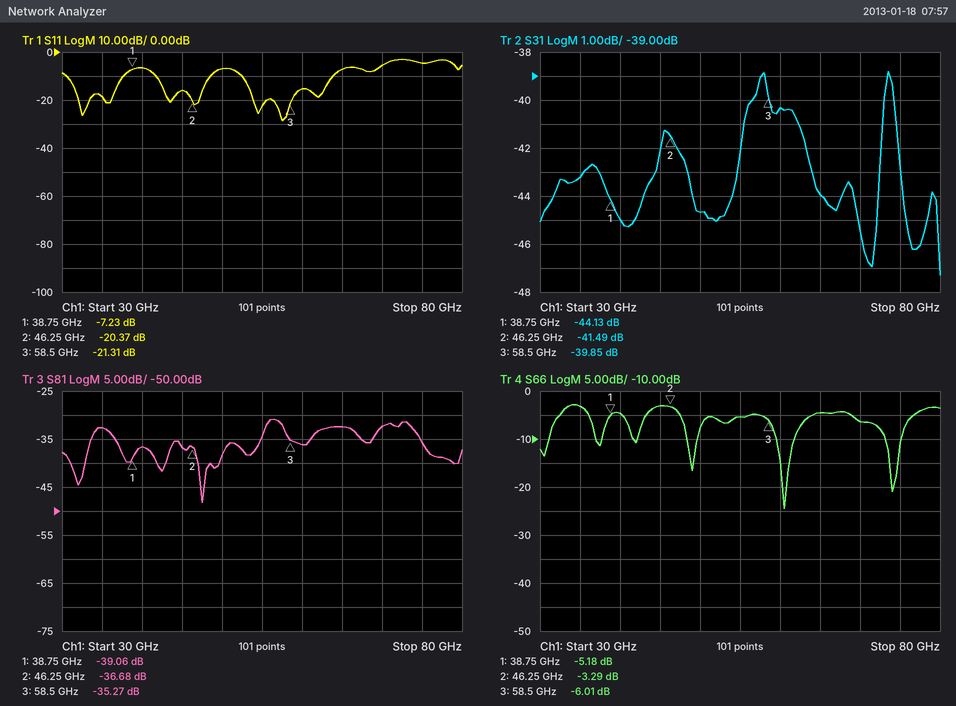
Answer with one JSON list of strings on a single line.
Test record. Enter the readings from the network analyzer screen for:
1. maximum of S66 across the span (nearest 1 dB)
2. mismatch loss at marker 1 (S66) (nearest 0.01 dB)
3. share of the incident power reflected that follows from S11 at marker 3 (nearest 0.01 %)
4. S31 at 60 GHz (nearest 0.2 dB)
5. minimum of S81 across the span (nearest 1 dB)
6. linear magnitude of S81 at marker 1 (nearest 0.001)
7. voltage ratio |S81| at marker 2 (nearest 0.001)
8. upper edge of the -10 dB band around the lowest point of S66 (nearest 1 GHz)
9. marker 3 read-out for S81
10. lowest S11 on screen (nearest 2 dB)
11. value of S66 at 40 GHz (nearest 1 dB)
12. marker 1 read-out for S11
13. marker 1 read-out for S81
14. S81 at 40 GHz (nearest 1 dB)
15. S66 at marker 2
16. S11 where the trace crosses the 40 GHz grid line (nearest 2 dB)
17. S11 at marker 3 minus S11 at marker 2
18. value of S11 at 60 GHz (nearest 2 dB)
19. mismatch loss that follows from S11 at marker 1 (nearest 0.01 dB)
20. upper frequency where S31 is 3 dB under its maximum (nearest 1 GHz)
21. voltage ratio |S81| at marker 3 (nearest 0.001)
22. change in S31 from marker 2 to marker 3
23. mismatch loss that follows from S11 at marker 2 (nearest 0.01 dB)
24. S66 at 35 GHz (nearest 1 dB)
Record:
["-3 dB", "1.57 dB", "0.74 %", "-40.4 dB", "-48 dB", "0.011", "0.015", "62 GHz", "-35.27 dB", "-28 dB", "-5 dB", "-7.23 dB", "-39.06 dB", "-37 dB", "-3.29 dB", "-6 dB", "-0.94 dB", "-16 dB", "0.91 dB", "75 GHz", "0.017", "1.64 dB", "0.04 dB", "-3 dB"]
